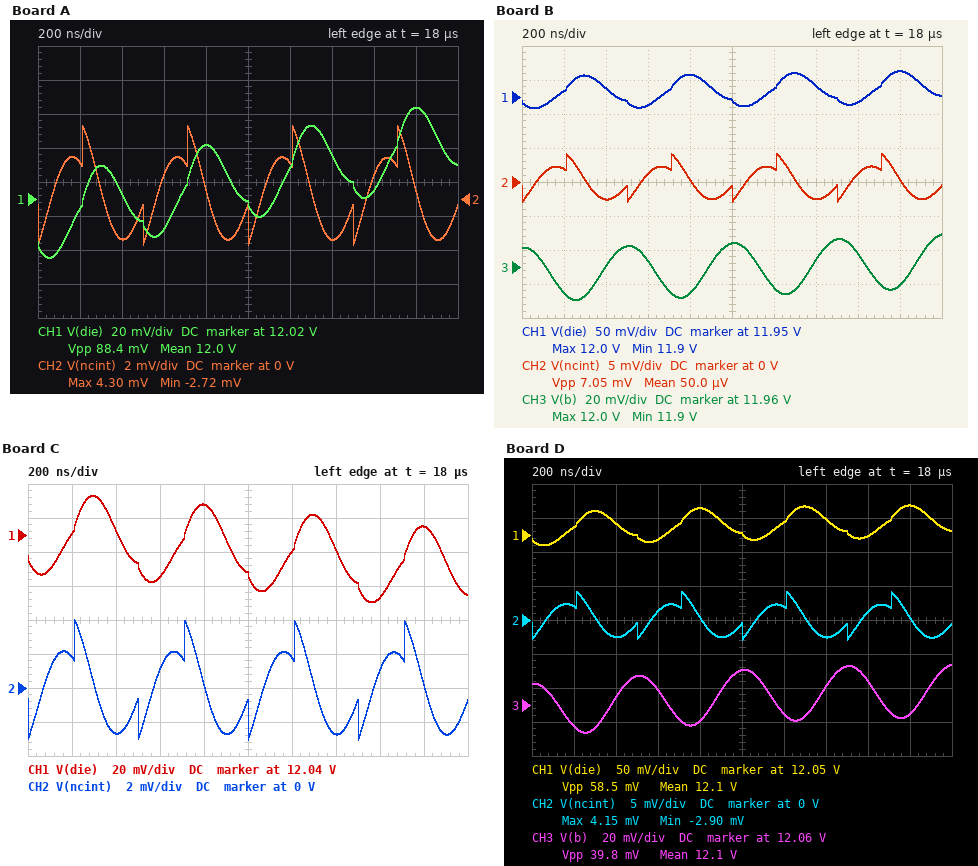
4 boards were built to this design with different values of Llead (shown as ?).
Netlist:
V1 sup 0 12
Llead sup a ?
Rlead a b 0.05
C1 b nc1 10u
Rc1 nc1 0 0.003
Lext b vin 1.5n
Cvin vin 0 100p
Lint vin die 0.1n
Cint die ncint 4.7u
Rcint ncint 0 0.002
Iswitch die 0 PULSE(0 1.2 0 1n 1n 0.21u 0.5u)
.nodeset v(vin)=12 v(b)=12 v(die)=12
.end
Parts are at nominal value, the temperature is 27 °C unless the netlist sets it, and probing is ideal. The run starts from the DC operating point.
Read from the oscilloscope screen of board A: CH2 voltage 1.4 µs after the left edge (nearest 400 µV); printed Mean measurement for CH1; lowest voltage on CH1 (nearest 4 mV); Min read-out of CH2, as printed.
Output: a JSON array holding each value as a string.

["-2.4 mV", "12.0 V", "11.984 V", "-2.72 mV"]
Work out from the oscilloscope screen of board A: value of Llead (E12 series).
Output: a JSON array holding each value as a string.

["1.8 µH"]
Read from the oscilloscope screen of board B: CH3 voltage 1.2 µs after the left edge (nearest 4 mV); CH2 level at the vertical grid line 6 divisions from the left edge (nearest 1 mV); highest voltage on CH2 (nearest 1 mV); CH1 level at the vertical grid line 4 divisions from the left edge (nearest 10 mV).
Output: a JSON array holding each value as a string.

["11.948 V", "2 mV", "4 mV", "11.98 V"]
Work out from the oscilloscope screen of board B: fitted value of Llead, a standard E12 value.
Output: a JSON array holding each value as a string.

["330 nH"]
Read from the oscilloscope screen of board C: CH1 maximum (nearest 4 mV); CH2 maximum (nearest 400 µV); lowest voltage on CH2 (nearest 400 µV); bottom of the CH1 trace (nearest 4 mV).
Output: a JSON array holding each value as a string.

["12.064 V", "4.0 mV", "-3.2 mV", "12.000 V"]
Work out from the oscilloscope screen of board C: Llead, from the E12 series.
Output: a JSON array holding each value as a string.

["820 nH"]
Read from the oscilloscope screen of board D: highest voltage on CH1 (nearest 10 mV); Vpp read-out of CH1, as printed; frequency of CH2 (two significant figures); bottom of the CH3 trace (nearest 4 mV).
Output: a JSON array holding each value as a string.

["12.09 V", "58.5 mV", "2.0 MHz", "12.044 V"]
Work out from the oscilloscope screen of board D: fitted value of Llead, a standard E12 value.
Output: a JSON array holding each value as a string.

["1.2 µH"]
